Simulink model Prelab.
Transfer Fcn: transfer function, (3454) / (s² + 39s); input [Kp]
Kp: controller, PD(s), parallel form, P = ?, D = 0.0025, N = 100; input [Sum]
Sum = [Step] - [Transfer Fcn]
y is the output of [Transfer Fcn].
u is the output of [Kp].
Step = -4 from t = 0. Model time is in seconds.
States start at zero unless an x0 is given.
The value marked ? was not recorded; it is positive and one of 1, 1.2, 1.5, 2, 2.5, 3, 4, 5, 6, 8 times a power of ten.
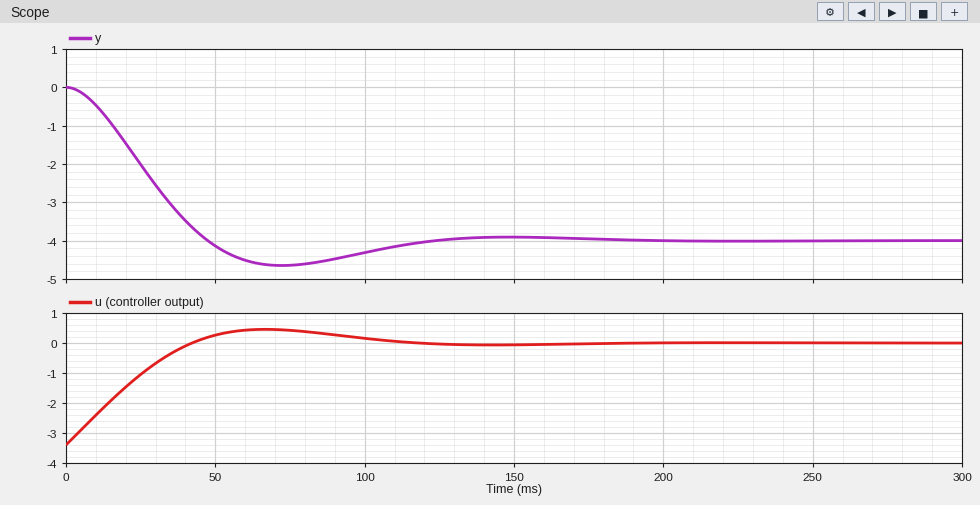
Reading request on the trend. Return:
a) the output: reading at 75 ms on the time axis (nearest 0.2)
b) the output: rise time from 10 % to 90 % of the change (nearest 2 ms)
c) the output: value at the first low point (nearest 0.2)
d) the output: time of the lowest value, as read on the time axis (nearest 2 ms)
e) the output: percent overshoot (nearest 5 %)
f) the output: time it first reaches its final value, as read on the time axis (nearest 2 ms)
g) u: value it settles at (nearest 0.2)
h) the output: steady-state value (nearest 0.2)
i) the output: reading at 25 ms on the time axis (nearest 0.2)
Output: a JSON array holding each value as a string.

["-4.6", "32 ms", "-4.6", "72 ms", "15 %", "48 ms", "0.0", "-4.0", "-2.0"]
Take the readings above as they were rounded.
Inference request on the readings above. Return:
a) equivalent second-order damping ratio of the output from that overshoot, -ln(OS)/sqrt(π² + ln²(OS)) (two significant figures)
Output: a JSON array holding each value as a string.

["0.52"]
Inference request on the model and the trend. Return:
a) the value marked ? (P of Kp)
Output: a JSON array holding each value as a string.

["0.6"]
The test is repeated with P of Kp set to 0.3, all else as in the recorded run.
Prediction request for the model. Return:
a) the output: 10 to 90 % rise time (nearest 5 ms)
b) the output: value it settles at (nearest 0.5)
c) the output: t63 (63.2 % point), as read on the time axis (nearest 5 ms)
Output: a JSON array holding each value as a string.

["60 ms", "-4.0", "45 ms"]
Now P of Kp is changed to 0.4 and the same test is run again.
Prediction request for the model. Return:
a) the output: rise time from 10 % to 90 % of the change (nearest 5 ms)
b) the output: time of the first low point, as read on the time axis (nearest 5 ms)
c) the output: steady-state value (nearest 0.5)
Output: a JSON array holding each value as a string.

["45 ms", "95 ms", "-4.0"]
